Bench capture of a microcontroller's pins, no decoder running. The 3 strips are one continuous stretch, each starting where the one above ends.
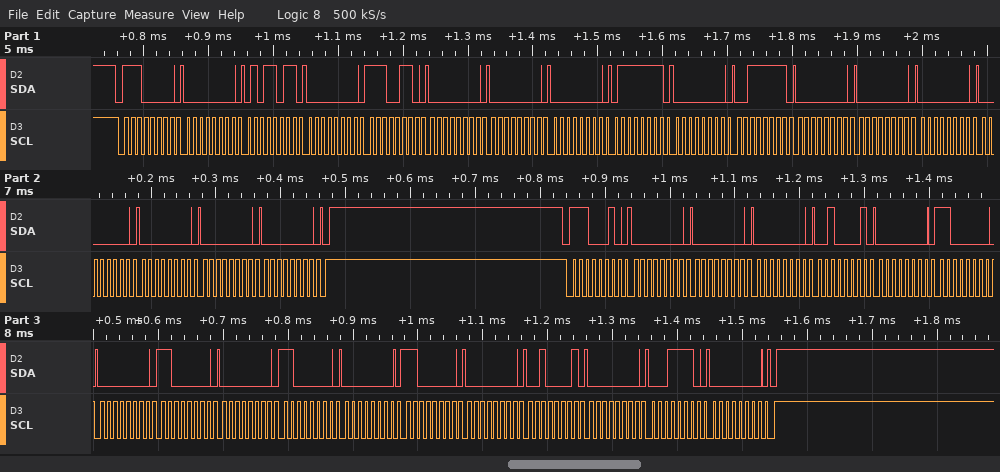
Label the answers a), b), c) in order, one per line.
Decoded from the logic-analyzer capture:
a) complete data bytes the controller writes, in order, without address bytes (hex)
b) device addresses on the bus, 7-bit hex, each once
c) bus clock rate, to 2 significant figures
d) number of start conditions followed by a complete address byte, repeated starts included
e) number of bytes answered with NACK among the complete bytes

a) 00 5B 00 E6 00 00 00 7F 00 3F 00 00 00 00 00 00 00 00 00 00 21 00 C0 00 C0 00 C0 00 C0 00 21 00 1E 00
b) 0x70 0x71
c) 100 kHz
d) 2
e) 0
